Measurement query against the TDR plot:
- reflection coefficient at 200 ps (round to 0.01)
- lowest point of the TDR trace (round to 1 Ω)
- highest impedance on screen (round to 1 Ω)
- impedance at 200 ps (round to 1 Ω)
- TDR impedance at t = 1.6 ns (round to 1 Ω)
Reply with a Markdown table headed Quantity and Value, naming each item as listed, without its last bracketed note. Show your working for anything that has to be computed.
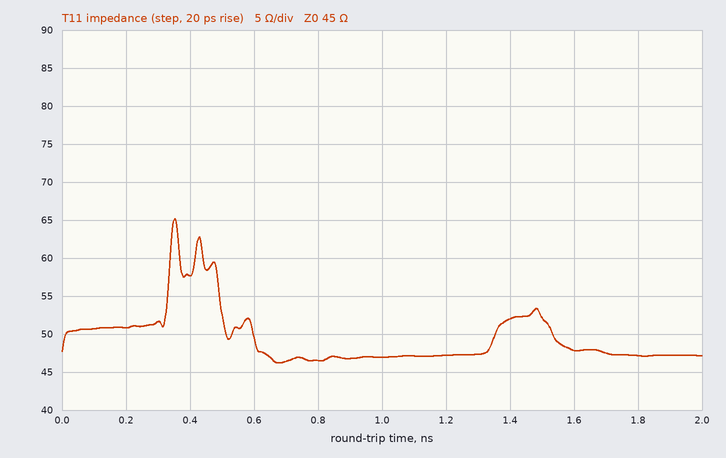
| Quantity | Value |
|---|---|
| reflection coefficient at 200 ps | (51 − 45)/(51 + 45) ≈ +0.06 |
| lowest point of the TDR trace | 46 Ω |
| highest impedance on screen | 65 Ω |
| impedance at 200 ps | 51 Ω |
| TDR impedance at t = 1.6 ns | 48 Ω |
